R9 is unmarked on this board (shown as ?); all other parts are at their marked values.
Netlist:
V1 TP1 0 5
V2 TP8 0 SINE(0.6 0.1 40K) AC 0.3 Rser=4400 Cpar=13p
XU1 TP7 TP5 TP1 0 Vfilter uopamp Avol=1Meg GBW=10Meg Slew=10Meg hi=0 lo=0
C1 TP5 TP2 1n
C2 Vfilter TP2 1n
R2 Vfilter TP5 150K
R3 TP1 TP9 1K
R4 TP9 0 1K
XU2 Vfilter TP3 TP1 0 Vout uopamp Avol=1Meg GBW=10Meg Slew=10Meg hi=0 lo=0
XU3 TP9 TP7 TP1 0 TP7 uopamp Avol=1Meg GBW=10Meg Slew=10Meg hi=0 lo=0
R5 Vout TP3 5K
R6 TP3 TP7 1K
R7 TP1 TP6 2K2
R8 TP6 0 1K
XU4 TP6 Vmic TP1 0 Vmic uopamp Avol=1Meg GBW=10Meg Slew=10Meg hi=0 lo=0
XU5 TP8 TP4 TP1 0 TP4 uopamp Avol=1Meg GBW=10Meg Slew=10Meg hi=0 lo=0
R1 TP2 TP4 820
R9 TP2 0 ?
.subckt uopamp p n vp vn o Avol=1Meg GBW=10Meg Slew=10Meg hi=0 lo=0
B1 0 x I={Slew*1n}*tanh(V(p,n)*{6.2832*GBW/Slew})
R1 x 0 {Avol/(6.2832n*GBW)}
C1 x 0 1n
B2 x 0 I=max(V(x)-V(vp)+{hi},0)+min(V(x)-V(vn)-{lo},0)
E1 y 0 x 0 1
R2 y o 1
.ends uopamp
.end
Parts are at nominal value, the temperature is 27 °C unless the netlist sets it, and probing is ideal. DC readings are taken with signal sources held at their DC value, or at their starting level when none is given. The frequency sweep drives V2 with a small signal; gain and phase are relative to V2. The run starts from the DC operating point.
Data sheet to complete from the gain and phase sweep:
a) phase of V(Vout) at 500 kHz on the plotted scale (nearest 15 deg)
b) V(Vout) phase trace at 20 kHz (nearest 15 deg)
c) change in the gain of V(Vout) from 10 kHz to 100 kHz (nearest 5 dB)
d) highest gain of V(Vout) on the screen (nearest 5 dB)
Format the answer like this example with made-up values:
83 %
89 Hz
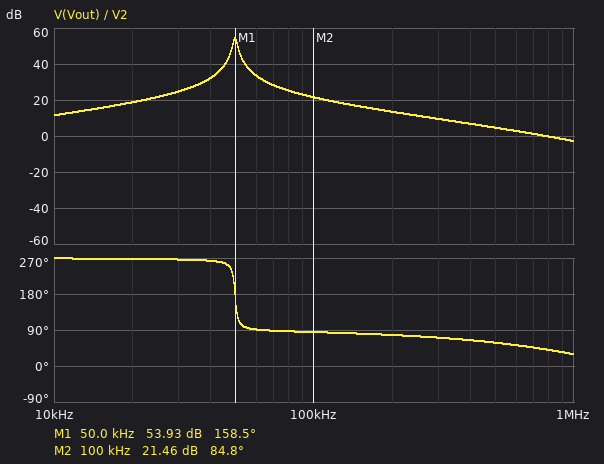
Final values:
60 deg
270 deg
10 dB
55 dB
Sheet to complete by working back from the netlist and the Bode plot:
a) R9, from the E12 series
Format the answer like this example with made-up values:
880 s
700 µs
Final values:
56 Ω
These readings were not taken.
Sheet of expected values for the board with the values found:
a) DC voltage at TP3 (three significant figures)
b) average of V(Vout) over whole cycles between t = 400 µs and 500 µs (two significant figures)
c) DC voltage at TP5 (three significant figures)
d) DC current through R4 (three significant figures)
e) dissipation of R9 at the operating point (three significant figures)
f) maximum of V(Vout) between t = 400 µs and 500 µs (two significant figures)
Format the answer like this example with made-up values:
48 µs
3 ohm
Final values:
2.50 V
2.5 V
2.50 V
2.50 mA
26.3 µW
5.0 V
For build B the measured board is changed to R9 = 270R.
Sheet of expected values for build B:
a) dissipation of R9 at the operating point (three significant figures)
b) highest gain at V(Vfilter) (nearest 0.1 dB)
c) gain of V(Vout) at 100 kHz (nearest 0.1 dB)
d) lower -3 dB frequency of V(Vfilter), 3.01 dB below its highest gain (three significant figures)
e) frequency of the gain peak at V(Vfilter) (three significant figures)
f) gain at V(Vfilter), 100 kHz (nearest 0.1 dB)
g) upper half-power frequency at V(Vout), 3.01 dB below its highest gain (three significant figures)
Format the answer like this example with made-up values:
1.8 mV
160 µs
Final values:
81.8 µW
39.2 dB
21.3 dB
26.8 kHz
27.8 kHz
5.8 dB
28.8 kHz
